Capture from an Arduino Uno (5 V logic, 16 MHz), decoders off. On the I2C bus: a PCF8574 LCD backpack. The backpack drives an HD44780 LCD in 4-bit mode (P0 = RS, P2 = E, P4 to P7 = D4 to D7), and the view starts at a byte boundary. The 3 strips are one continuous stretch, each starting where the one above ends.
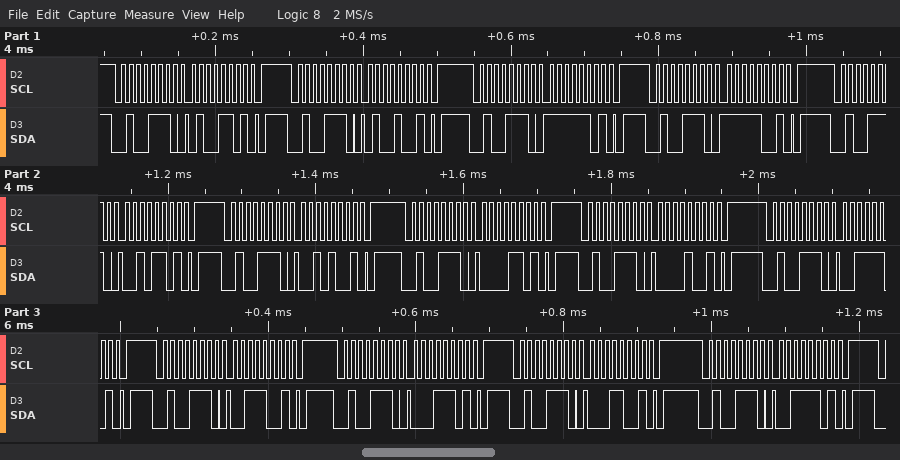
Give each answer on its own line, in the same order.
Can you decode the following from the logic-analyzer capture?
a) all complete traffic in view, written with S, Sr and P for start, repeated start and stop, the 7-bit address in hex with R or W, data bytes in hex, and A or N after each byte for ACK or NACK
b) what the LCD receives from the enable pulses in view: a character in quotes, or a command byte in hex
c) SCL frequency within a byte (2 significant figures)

S 27W A 4D A P S 27W A 49 A P S 27W A FD A P S 27W A F9 A P S 27W A 2D A P S 27W A 29 A P S 27W A 0D A P S 27W A 09 A P S 27W A 3D A P S 27W A 39 A P S 27W A 1D A P S 27W A 19 A P S 27W A 3D A P
'O' ' ' '1'
100 kHz
